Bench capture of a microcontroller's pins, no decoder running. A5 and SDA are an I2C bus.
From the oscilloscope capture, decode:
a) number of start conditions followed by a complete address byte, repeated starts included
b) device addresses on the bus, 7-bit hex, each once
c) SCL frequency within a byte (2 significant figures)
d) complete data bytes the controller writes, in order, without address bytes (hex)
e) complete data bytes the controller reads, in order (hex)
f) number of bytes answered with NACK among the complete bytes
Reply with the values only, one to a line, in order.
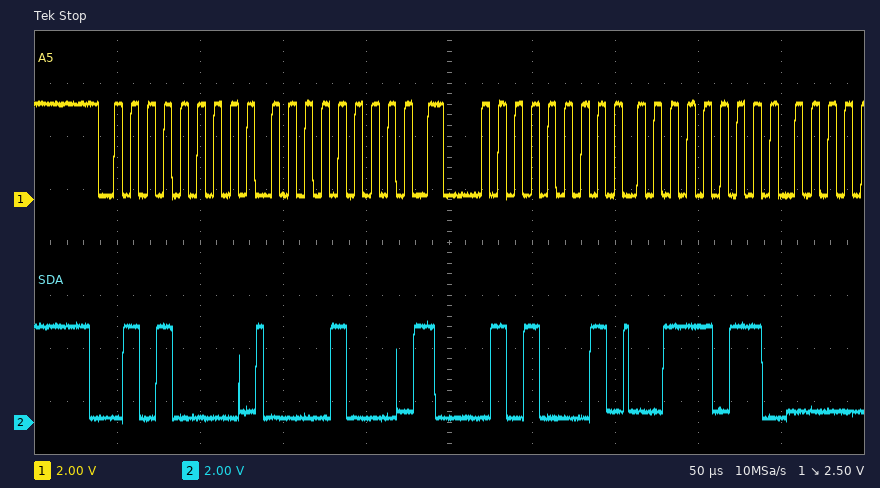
2
0x28
100 kHz
08
3B
0
